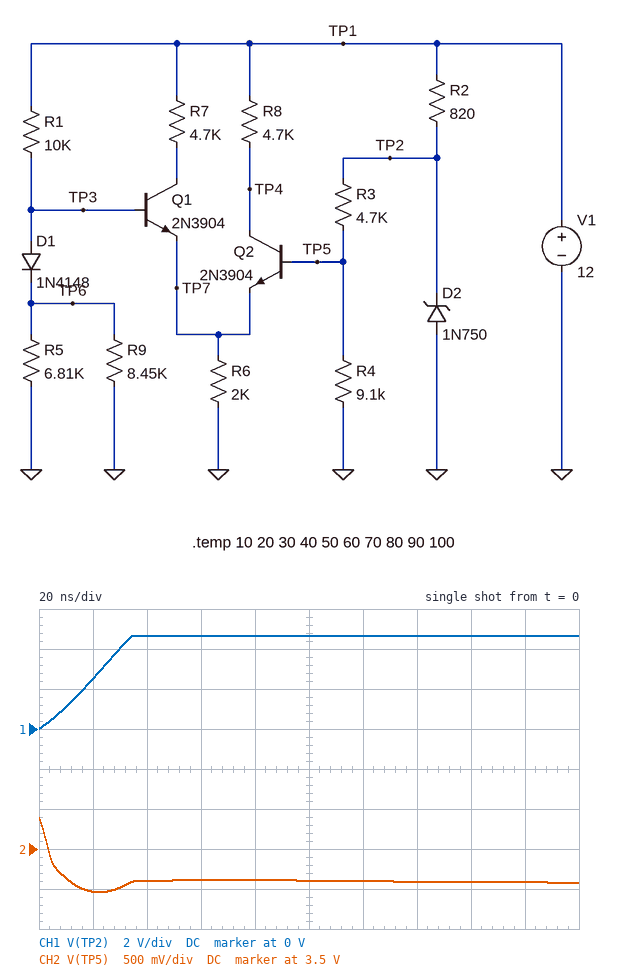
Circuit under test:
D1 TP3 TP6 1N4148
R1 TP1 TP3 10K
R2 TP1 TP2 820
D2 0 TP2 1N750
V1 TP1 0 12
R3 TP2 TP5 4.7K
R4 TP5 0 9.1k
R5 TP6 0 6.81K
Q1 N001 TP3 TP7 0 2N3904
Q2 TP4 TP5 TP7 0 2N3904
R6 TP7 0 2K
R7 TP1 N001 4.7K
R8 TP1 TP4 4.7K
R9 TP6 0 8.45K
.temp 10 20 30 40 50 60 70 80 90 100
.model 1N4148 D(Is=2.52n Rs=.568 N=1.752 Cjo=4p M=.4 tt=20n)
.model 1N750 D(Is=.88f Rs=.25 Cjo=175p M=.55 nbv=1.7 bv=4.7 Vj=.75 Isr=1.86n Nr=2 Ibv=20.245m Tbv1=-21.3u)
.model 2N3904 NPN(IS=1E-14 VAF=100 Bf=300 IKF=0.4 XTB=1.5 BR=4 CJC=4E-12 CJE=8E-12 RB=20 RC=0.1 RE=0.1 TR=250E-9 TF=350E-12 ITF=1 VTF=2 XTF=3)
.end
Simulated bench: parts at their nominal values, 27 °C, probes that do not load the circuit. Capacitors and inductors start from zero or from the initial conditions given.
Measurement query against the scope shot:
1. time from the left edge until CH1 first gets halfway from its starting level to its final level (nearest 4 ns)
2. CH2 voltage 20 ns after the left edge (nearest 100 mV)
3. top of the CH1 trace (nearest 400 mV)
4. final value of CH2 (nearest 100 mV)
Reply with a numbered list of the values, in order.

1. 20 ns
2. 3.0 V
3. 4.8 V
4. 3.1 V
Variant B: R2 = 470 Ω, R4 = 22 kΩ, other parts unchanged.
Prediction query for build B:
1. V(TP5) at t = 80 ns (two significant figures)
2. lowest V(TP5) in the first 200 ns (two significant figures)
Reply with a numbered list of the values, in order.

1. 3.8 V
2. 3.5 V
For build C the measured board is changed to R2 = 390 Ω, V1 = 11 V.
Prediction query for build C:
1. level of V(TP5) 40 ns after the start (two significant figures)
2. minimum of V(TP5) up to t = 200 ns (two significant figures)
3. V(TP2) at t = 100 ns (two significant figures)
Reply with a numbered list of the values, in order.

1. 3.2 V
2. 3.1 V
3. 4.7 V
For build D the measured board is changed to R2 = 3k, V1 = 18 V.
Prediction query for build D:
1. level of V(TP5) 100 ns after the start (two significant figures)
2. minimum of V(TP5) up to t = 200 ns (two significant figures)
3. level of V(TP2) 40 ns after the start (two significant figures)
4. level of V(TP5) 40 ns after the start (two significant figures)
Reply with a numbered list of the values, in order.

1. 2.9 V
2. 2.4 V
3. 2.2 V
4. 2.7 V
